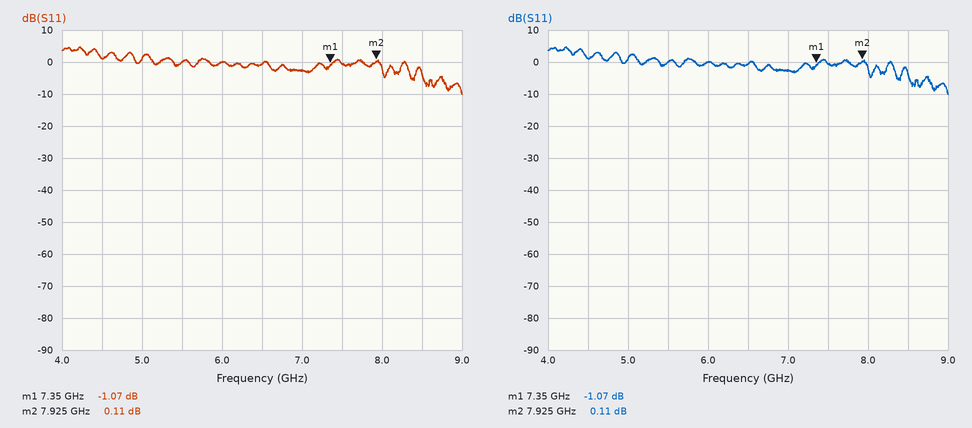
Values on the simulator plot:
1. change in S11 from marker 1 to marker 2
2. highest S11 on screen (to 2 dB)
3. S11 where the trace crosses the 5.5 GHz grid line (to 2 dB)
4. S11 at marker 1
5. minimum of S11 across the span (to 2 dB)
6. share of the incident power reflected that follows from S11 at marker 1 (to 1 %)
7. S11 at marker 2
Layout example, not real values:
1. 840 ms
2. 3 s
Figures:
1. 1.18 dB
2. 4 dB
3. 0 dB
4. -1.07 dB
5. -10 dB
6. 78 %
7. 0.11 dB
